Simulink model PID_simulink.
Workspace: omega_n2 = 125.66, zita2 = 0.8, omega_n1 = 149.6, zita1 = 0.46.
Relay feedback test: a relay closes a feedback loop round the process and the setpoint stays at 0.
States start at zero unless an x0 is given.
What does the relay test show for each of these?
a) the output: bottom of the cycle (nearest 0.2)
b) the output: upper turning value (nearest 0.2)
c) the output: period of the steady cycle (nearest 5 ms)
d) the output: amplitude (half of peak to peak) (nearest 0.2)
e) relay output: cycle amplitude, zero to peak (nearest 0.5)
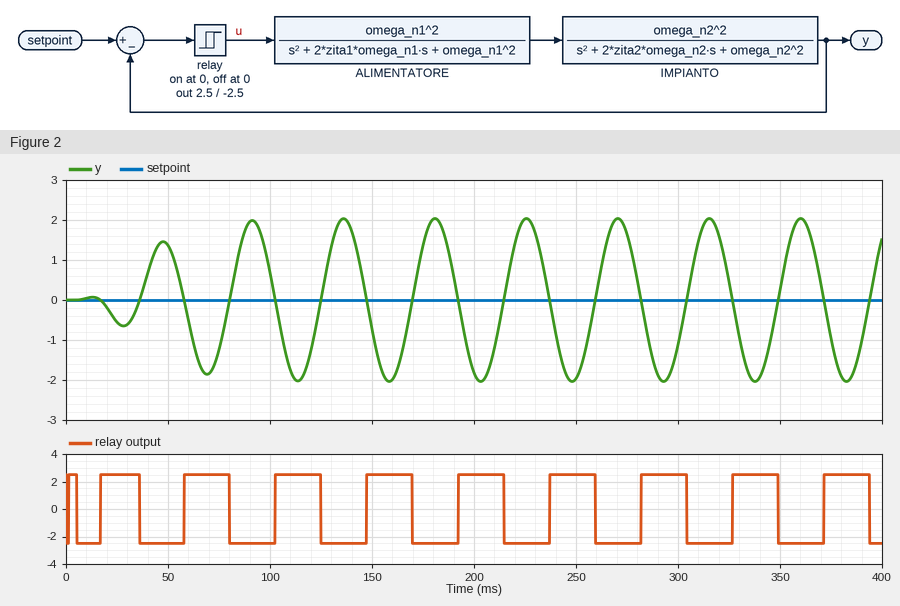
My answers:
-2.0
2.0
45 ms
2.0
2.5
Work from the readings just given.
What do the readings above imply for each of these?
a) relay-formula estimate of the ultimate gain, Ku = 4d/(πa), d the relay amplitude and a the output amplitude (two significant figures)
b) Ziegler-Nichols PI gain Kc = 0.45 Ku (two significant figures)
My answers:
1.6
0.72
